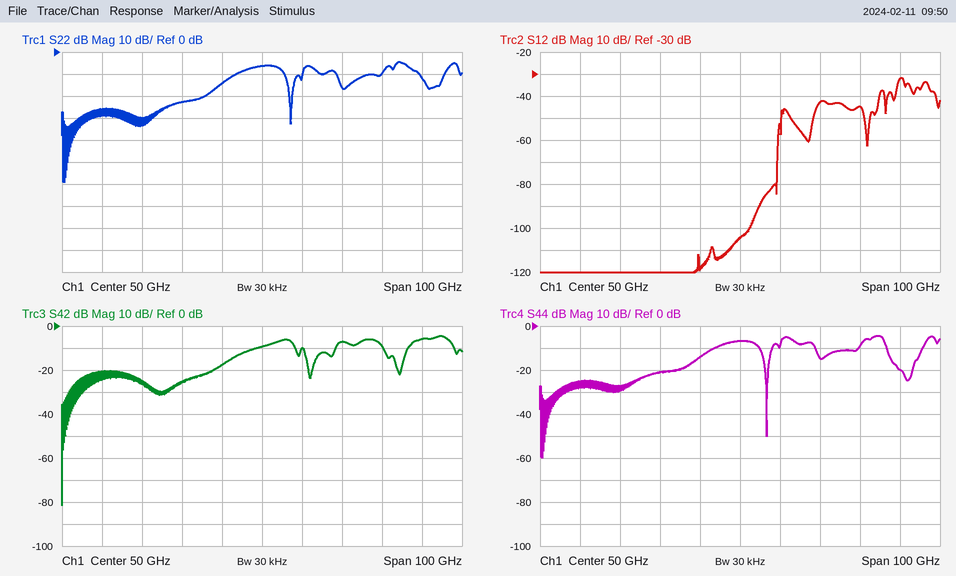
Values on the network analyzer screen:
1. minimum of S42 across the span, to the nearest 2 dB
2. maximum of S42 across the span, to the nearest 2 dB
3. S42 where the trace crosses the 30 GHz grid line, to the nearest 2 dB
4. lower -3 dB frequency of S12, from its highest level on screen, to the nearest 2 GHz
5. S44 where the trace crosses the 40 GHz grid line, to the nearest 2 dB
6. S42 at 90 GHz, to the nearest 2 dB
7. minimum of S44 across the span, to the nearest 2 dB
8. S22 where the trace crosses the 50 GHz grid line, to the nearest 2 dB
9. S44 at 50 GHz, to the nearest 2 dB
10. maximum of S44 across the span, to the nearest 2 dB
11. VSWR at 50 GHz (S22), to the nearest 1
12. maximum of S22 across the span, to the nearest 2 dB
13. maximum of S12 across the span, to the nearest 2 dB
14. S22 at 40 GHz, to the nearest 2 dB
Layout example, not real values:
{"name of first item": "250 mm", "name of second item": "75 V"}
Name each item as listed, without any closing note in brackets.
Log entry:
{"minimum of S42 across the span, to the nearest 2 dB": "-82 dB", "maximum of S42 across the span, to the nearest 2 dB": "-4 dB", "S42 where the trace crosses the 30 GHz grid line, to the nearest 2 dB": "-26 dB", "lower -3 dB frequency of S12, from its highest level on screen, to the nearest 2 GHz": "90 GHz", "S44 where the trace crosses the 40 GHz grid line, to the nearest 2 dB": "-14 dB", "S42 at 90 GHz, to the nearest 2 dB": "-6 dB", "minimum of S44 across the span, to the nearest 2 dB": "-60 dB", "S22 where the trace crosses the 50 GHz grid line, to the nearest 2 dB": "-6 dB", "S44 at 50 GHz, to the nearest 2 dB": "-6 dB", "maximum of S44 across the span, to the nearest 2 dB": "-4 dB", "VSWR at 50 GHz (S22), to the nearest 1": "3", "maximum of S22 across the span, to the nearest 2 dB": "-4 dB", "maximum of S12 across the span, to the nearest 2 dB": "-32 dB", "S22 at 40 GHz, to the nearest 2 dB": "-14 dB"}
